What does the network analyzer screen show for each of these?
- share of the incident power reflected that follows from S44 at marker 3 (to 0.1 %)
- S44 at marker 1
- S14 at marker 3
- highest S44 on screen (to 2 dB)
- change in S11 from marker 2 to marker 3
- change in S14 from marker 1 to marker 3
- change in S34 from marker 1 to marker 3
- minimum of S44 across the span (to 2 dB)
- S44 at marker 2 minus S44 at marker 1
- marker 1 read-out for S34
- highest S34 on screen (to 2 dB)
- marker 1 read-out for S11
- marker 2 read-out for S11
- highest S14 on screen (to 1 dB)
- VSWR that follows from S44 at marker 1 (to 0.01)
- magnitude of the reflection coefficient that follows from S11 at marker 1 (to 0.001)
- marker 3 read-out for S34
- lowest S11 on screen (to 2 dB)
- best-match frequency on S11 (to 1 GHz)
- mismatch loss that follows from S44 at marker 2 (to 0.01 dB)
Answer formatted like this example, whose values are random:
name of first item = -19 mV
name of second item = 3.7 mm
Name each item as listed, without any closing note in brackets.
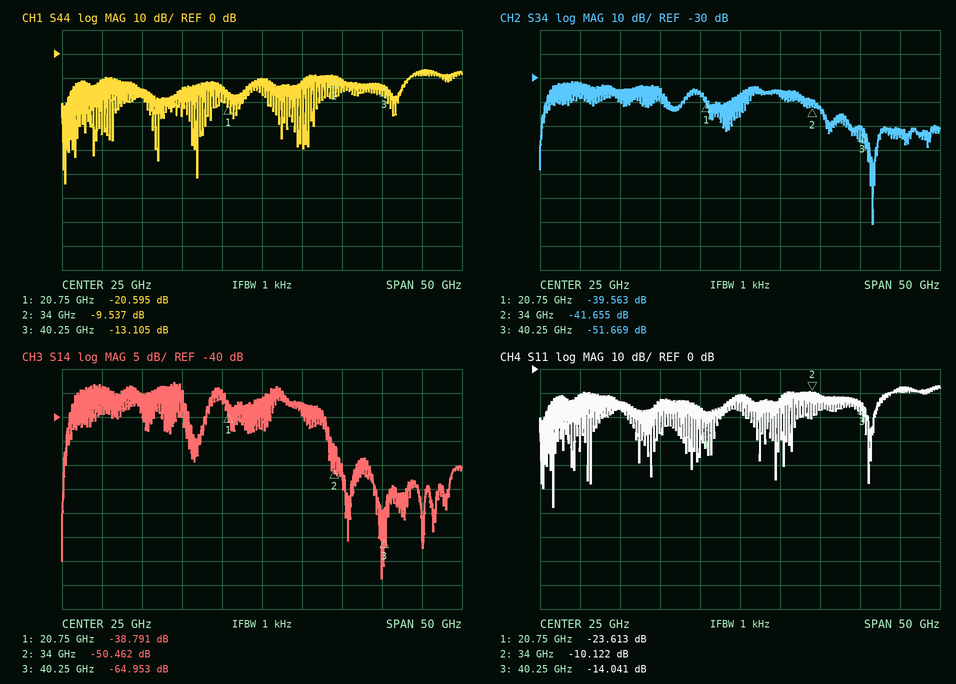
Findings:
share of the incident power reflected that follows from S44 at marker 3 = 4.9 %
S44 at marker 1 = -20.595 dB
S14 at marker 3 = -64.953 dB
highest S44 on screen = -6 dB
change in S11 from marker 2 to marker 3 = -3.919 dB
change in S14 from marker 1 to marker 3 = -26.162 dB
change in S34 from marker 1 to marker 3 = -12.106 dB
minimum of S44 across the span = -54 dB
S44 at marker 2 minus S44 at marker 1 = 11.058 dB
marker 1 read-out for S34 = -39.563 dB
highest S34 on screen = -32 dB
marker 1 read-out for S11 = -23.613 dB
marker 2 read-out for S11 = -10.122 dB
highest S14 on screen = -33 dB
VSWR that follows from S44 at marker 1 = 1.21
magnitude of the reflection coefficient that follows from S11 at marker 1 = 0.066
marker 3 read-out for S34 = -51.669 dB
lowest S11 on screen = -58 dB
best-match frequency on S11 = 2 GHz
mismatch loss that follows from S44 at marker 2 = 0.51 dB
